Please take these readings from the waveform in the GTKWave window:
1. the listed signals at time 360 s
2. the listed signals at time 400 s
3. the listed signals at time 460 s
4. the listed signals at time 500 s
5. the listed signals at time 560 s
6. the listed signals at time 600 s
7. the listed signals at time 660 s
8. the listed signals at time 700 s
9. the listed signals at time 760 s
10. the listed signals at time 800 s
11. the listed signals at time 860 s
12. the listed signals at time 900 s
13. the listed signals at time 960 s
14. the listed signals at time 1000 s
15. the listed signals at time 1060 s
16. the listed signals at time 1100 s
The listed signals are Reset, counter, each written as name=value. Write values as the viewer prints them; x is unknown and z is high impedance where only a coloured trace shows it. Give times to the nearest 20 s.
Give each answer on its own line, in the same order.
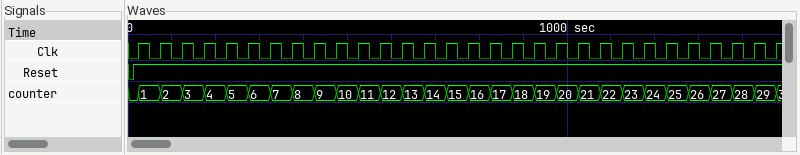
Reset=1, counter=7
Reset=1, counter=8
Reset=1, counter=9
Reset=1, counter=10
Reset=1, counter=11
Reset=1, counter=12
Reset=1, counter=13
Reset=1, counter=14
Reset=1, counter=15
Reset=1, counter=16
Reset=1, counter=17
Reset=1, counter=18
Reset=1, counter=19
Reset=1, counter=20
Reset=1, counter=21
Reset=1, counter=22
